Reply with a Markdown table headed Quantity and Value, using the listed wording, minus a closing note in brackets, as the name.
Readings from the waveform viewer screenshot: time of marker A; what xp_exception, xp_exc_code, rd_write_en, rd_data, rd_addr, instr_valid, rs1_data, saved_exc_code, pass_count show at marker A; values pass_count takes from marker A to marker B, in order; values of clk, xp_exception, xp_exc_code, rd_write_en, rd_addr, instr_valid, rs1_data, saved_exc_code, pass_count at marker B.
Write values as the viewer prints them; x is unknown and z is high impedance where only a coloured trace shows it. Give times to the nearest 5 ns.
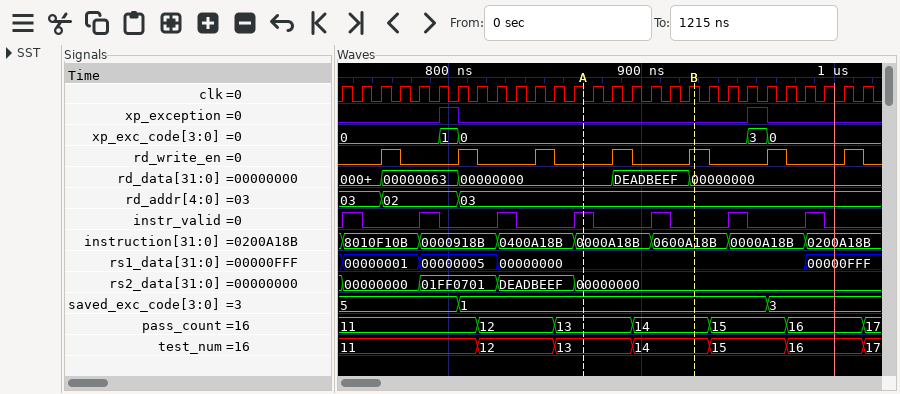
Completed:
| Quantity | Value |
|---|---|
| time of marker A | 870 ns |
| what xp_exception, xp_exc_code, rd_write_en, rd_data, rd_addr, instr_valid, rs1_data, saved_exc_code, pass_count show at marker A | xp_exception=0, xp_exc_code=0, rd_write_en=0, rd_data=00000000, rd_addr=03, instr_valid=1, rs1_data=00000000, saved_exc_code=1, pass_count=13 |
| values pass_count takes from marker A to marker B, in order | 13, 14 |
| values of clk, xp_exception, xp_exc_code, rd_write_en, rd_addr, instr_valid, rs1_data, saved_exc_code, pass_count at marker B | clk=1, xp_exception=0, xp_exc_code=0, rd_write_en=1, rd_addr=03, instr_valid=0, rs1_data=00000000, saved_exc_code=1, pass_count=14 |
